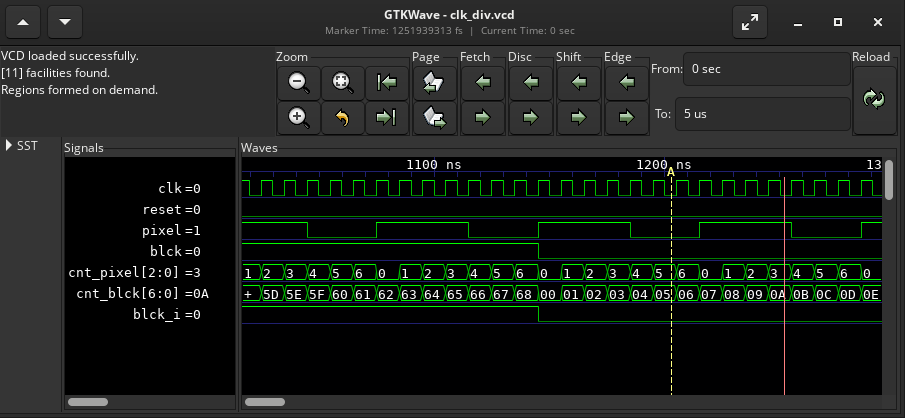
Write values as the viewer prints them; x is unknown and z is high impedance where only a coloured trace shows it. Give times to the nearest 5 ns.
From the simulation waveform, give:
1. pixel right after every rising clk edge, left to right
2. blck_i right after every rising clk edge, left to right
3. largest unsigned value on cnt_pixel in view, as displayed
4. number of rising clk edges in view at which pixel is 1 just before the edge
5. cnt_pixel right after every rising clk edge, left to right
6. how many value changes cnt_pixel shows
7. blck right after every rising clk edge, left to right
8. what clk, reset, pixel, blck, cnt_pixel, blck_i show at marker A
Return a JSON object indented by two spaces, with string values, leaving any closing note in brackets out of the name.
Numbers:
{
  "pixel right after every rising clk edge, left to right": "1 1 0 0 0 1 1 1 1 0 0 0 1 1 1 1 0 0 0 1 1 1 1 0 0 0 1",
  "blck_i right after every rising clk edge, left to right": "1 1 1 1 1 1 1 1 1 1 1 1 0 0 0 0 0 0 0 0 0 0 0 0 0 0 0",
  "largest unsigned value on cnt_pixel in view, as displayed": "6",
  "number of rising clk edges in view at which pixel is 1 just before the edge": "15",
  "cnt_pixel right after every rising clk edge, left to right": "2, 3, 4, 5, 6, 0, 1, 2, 3, 4, 5, 6, 0, 1, 2, 3, 4, 5, 6, 0, 1, 2, 3, 4, 5, 6, 0",
  "how many value changes cnt_pixel shows": "27",
  "blck right after every rising clk edge, left to right": "1 1 1 1 1 1 1 1 1 1 1 1 0 0 0 0 0 0 0 0 0 0 0 0 0 0 0",
  "what clk, reset, pixel, blck, cnt_pixel, blck_i show at marker A": "clk=0, reset=0, pixel=0, blck=0, cnt_pixel=5, blck_i=0"
}
